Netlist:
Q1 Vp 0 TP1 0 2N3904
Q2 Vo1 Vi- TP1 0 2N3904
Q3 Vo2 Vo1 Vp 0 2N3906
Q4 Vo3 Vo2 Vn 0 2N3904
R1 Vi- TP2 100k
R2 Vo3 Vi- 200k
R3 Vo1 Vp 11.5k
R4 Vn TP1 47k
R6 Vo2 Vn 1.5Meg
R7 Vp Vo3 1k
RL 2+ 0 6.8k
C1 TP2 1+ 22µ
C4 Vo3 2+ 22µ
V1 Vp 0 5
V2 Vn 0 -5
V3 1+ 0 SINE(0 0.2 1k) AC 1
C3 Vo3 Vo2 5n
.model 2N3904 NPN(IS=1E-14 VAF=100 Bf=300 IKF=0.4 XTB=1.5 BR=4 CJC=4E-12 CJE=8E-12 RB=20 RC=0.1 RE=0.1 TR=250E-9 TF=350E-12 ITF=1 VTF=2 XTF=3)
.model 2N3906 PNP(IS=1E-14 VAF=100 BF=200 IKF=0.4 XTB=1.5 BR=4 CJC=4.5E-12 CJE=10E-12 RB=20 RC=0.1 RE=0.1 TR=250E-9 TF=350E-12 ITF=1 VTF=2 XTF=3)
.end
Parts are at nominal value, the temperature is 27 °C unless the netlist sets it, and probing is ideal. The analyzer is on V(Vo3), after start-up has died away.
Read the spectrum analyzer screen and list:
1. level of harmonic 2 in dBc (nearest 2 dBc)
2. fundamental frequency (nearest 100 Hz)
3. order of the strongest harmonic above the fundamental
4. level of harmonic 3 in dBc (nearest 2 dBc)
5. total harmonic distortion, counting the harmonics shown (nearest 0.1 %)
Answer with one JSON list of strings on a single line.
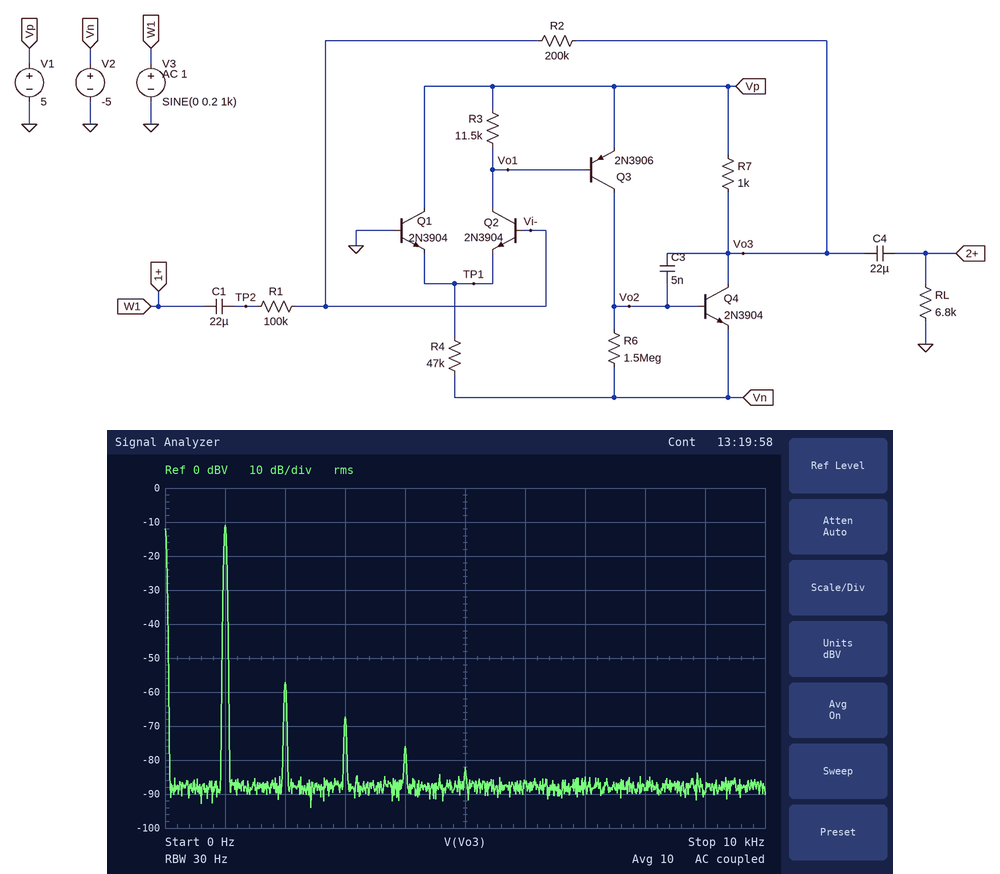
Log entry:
["-46 dBc", "1.0 kHz", "2", "-56 dBc", "0.5 %"]
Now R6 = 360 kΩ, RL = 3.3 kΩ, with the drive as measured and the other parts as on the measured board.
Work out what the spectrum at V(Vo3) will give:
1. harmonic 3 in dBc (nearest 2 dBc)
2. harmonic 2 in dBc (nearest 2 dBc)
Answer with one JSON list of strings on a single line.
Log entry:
["-60 dBc", "-48 dBc"]
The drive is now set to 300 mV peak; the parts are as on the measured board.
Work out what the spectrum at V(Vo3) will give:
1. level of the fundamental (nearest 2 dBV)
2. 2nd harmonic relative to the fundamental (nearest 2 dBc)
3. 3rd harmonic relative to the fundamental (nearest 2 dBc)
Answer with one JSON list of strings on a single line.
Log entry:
["-8 dBV", "-30 dBc", "-34 dBc"]
